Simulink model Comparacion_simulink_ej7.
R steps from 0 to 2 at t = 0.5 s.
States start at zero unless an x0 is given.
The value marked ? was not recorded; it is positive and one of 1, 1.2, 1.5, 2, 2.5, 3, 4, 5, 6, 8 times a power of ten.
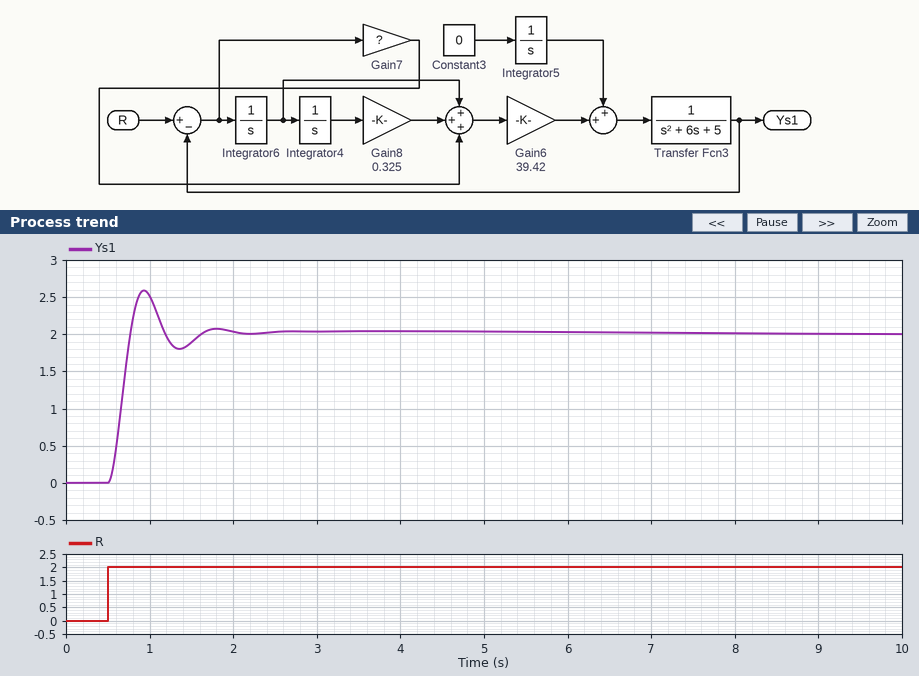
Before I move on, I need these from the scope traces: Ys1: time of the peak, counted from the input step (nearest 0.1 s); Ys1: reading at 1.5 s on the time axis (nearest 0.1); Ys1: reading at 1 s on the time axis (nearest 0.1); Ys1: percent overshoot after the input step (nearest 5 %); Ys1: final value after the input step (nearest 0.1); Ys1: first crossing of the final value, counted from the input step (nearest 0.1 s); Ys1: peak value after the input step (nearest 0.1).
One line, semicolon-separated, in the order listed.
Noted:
0.4 s; 1.9; 2.5; 30 %; 2.0; 0.3 s; 2.6
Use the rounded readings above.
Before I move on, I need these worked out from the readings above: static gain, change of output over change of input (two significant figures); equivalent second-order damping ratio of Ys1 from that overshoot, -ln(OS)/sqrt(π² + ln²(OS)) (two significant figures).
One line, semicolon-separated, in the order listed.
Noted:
1.0; 0.36
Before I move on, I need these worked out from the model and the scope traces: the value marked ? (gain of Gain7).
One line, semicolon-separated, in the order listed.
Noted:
1.5
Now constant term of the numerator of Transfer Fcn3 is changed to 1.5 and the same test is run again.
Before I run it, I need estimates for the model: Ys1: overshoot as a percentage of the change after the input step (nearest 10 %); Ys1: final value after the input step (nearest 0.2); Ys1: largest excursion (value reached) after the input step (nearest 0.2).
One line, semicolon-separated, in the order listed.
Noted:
40 %; 2.0; 2.8
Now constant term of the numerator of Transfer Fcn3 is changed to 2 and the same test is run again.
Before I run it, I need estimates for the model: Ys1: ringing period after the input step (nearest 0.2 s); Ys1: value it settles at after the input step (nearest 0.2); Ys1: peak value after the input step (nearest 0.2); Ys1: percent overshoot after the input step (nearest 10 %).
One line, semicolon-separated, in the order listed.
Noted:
0.6 s; 2.0; 2.8; 40 %
